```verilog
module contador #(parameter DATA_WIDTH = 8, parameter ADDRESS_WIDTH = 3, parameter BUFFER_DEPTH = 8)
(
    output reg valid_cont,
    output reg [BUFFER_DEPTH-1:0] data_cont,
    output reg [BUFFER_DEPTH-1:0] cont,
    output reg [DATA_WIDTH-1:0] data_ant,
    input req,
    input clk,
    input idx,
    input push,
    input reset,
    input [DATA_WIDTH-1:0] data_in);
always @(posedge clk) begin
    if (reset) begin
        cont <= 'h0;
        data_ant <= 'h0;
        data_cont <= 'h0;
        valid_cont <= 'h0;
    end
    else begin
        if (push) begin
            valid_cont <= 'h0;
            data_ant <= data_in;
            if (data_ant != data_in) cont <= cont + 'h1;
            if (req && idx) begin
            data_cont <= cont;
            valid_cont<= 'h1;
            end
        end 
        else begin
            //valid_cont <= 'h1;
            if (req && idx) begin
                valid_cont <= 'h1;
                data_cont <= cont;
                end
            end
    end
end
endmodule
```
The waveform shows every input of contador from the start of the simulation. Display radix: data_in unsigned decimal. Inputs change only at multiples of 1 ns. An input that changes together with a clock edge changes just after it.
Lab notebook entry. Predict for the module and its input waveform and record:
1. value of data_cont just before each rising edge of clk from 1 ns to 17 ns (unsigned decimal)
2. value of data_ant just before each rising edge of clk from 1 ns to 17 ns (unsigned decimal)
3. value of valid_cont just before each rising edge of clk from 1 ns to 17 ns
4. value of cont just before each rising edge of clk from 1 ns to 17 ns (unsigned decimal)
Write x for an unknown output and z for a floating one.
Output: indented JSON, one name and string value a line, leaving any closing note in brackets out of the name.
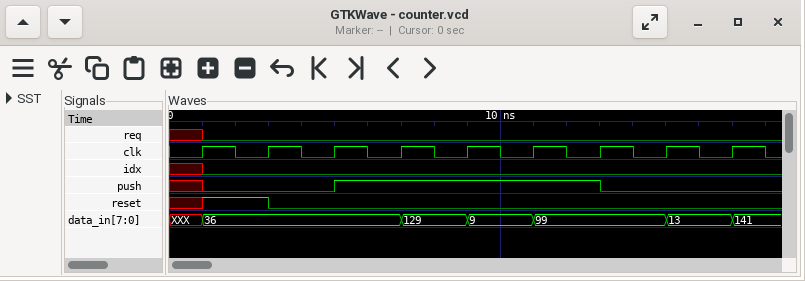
{
  "value of data_cont just before each rising edge of clk from 1 ns to 17 ns": "x, x, 0, 0, 0, 0, 0, 0, 0",
  "value of data_ant just before each rising edge of clk from 1 ns to 17 ns": "x, x, 0, 0, 36, 129, 9, 99, 99",
  "value of valid_cont just before each rising edge of clk from 1 ns to 17 ns": "x x 0 0 0 0 0 0 0",
  "value of cont just before each rising edge of clk from 1 ns to 17 ns": "x, x, 0, 0, 1, 2, 3, 4, 4"
}
